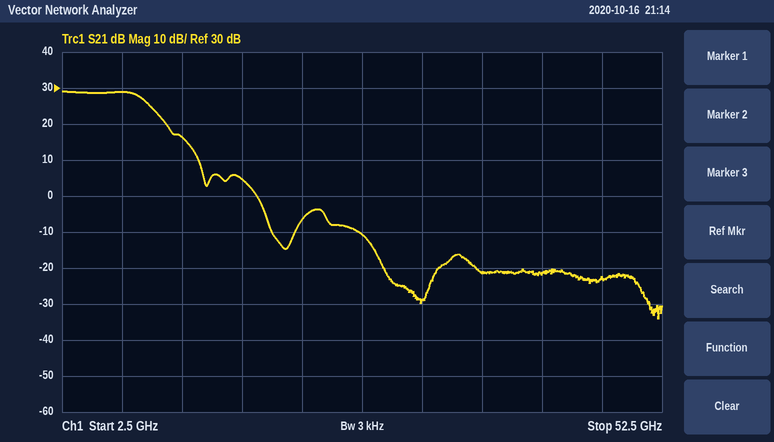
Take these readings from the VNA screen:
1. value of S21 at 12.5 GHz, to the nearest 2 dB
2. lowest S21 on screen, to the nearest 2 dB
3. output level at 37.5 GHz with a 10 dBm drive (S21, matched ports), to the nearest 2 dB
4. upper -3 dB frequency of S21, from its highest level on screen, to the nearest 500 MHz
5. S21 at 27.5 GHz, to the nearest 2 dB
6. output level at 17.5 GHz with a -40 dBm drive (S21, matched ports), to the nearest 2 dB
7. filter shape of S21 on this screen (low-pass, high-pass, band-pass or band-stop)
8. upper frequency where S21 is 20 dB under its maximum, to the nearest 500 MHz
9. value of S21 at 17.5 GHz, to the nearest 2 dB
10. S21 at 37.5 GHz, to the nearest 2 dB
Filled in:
16 dB
-34 dB
-12 dBm
9.5 GHz
-10 dB
-36 dBm
low-pass
14.0 GHz
4 dB
-22 dB
